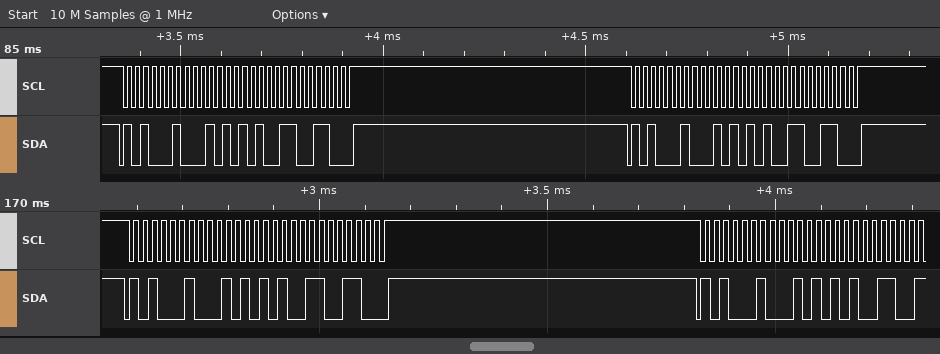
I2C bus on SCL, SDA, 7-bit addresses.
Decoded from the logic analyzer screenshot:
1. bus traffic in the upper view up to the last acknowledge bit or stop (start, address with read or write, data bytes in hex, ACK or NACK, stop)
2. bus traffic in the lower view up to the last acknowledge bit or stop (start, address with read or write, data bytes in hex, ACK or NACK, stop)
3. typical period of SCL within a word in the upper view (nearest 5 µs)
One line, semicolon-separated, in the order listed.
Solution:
start, address 51 write ACK, 55 ACK, 66 ACK, stop, start, address 51 write ACK, 55 ACK, 66 ACK, stop; start, address 51 write ACK, 55 ACK, 66 ACK, stop, start, address 51 write ACK, 55 ACK; 20 µs
